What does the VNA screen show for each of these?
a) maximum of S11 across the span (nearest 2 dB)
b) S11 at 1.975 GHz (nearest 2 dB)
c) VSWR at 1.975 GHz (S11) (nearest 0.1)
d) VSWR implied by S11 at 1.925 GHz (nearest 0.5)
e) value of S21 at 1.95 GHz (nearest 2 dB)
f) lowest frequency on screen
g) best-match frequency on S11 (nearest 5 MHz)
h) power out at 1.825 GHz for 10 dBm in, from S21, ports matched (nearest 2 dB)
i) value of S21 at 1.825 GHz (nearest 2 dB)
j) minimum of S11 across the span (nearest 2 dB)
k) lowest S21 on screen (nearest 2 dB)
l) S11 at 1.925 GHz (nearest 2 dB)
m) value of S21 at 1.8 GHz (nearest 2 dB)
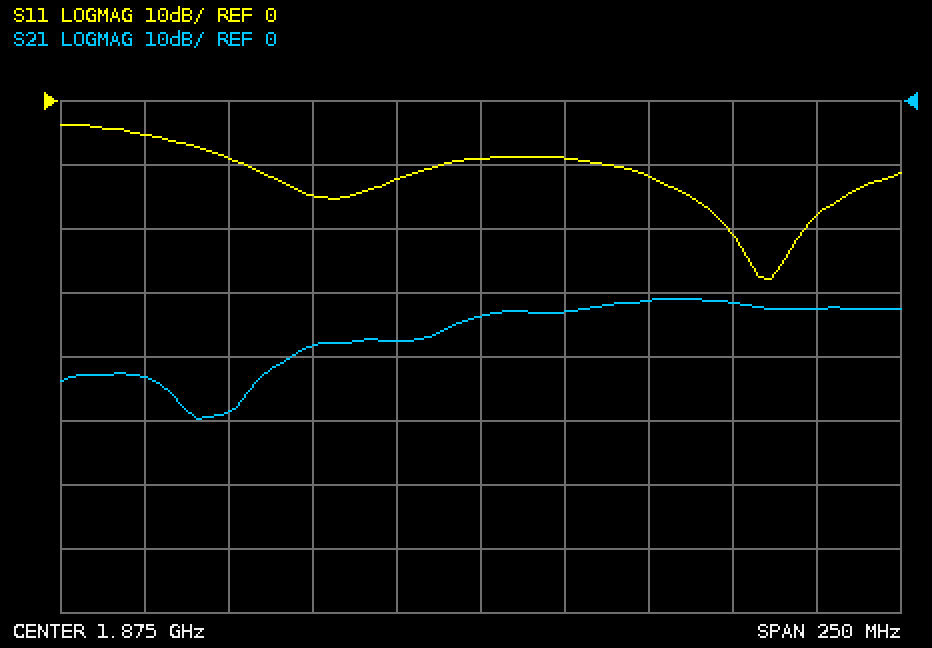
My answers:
-4 dB
-18 dB
1.3
1.5
-32 dB
1.75 GHz
1.960 GHz
-28 dBm
-38 dB
-28 dB
-50 dB
-12 dB
-48 dB
